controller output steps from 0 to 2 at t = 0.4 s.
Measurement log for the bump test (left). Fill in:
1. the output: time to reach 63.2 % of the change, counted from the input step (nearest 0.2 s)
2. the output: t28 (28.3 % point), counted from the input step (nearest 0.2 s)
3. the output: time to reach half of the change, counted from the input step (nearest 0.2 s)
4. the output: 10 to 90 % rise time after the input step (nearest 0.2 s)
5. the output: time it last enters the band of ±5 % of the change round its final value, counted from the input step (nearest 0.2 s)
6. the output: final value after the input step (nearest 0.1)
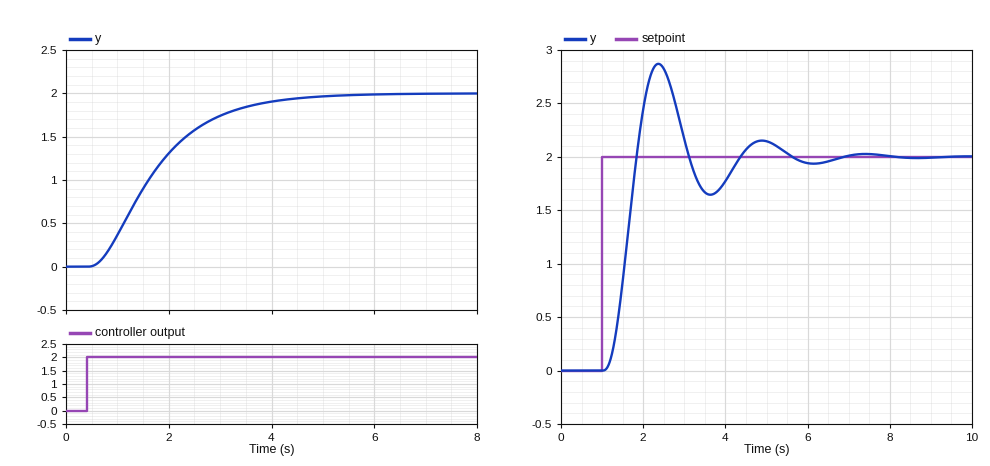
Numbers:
1.6 s
0.8 s
1.2 s
2.4 s
3.6 s
2.0
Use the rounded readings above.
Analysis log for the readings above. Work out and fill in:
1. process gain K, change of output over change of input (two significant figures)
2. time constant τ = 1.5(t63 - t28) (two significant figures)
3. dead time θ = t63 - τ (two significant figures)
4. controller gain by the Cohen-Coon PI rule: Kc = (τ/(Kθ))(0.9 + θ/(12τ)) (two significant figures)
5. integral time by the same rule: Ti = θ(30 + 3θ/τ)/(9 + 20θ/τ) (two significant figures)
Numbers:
1.0
1.2 s
0.40 s
2.8
0.79 s
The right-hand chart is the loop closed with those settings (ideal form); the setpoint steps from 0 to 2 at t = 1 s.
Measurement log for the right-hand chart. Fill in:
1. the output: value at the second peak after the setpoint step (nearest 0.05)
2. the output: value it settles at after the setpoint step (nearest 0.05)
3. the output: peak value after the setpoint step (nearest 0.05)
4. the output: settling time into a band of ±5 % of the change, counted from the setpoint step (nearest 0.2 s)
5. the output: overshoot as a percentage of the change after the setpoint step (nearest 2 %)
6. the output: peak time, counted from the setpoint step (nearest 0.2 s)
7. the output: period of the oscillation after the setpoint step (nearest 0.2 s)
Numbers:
2.15
2.00
2.85
4.2 s
44 %
1.4 s
2.6 s
